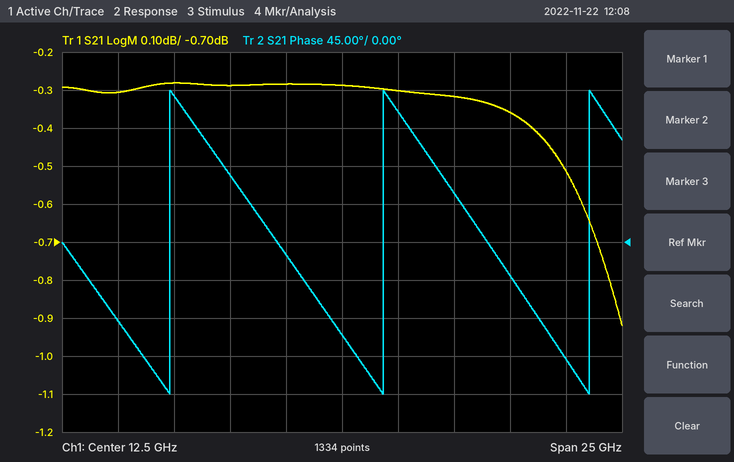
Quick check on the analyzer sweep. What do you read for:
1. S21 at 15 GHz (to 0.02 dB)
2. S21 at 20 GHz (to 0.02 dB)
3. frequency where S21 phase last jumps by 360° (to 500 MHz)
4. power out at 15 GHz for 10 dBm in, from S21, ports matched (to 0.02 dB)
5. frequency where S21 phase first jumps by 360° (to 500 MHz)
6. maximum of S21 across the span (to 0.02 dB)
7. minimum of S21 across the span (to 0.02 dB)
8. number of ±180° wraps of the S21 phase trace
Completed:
-0.30 dB
-0.36 dB
23.5 GHz
9.70 dBm
5.0 GHz
-0.28 dB
-0.92 dB
3
